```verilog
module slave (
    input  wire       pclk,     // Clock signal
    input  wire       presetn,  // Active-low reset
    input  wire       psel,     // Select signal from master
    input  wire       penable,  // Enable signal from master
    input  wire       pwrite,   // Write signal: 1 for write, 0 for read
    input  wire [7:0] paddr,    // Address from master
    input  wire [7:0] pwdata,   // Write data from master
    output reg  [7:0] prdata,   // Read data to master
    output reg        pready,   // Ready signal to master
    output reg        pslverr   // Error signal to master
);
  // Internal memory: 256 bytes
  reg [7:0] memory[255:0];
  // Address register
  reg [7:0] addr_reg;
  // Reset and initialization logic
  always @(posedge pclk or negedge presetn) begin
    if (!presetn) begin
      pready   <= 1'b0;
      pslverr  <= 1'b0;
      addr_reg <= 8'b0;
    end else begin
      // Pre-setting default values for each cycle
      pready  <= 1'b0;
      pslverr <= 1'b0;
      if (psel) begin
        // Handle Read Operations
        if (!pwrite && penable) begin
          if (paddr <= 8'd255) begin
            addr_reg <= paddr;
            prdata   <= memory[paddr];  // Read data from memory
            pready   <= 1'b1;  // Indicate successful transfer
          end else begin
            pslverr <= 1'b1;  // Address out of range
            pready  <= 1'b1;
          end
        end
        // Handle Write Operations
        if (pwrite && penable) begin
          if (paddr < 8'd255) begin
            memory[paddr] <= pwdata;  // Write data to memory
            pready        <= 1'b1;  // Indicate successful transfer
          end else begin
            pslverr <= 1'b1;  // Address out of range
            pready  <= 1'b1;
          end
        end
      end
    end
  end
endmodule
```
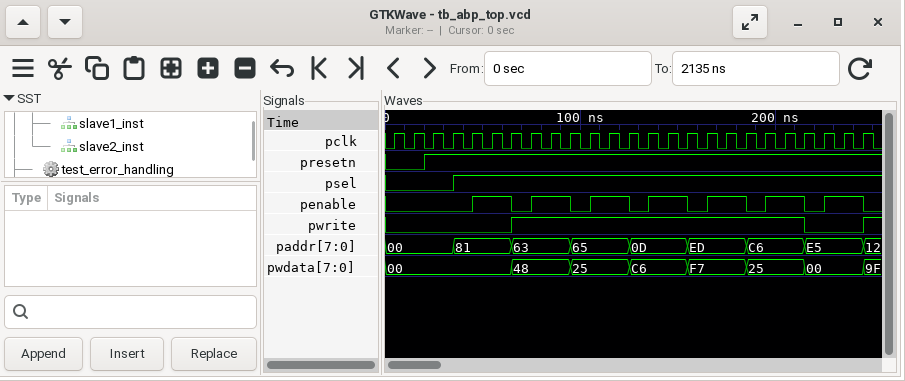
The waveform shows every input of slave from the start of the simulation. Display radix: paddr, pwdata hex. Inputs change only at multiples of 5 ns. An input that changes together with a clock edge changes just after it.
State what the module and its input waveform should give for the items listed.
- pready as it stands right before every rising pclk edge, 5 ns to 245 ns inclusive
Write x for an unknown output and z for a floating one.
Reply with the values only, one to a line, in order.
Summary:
0 0 0 0 0 0 1 1 0 1 1 0 1 1 0 1 1 0 1 1 0 1 1 0 1
